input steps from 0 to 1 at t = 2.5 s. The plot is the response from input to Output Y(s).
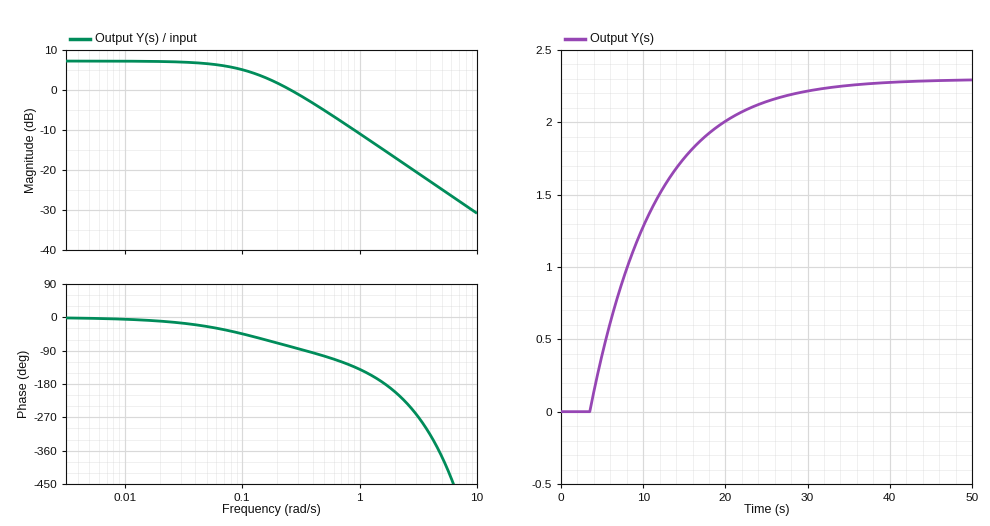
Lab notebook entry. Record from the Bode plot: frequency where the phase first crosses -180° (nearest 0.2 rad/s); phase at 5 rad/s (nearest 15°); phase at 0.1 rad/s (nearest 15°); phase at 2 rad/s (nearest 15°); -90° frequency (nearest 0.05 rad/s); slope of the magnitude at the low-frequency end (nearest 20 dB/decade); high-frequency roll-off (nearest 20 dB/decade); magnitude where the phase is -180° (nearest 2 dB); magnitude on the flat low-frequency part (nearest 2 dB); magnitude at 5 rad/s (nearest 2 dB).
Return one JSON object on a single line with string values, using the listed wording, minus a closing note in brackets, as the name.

{"frequency where the phase first crosses -180°": "1.6 rad/s", "phase at 5 rad/s": "-375°", "phase at 0.1 rad/s": "-45°", "phase at 2 rad/s": "-195°", "-90° frequency": "0.35 rad/s", "slope of the magnitude at the low-frequency end": "0 dB/decade", "high-frequency roll-off": "-20 dB/decade", "magnitude where the phase is -180°": "-16 dB", "magnitude on the flat low-frequency part": "8 dB", "magnitude at 5 rad/s": "-24 dB"}
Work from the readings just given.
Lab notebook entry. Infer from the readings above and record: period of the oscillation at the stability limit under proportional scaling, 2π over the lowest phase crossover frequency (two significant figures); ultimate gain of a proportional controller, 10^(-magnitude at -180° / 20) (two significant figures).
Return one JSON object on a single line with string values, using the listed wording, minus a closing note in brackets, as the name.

{"period of the oscillation at the stability limit under proportional scaling, 2π over the lowest phase crossover frequency": "3.9 s", "ultimate gain of a proportional controller, 10^(-magnitude at -180° / 20)": "6.3"}
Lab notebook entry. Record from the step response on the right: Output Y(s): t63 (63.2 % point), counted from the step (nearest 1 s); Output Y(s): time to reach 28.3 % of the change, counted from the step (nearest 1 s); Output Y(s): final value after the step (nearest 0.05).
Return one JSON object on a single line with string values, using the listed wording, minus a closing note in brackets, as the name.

{"Output Y(s): t63 (63.2 % point), counted from the step": "9 s", "Output Y(s): time to reach 28.3 % of the change, counted from the step": "4 s", "Output Y(s): final value after the step": "2.30"}
